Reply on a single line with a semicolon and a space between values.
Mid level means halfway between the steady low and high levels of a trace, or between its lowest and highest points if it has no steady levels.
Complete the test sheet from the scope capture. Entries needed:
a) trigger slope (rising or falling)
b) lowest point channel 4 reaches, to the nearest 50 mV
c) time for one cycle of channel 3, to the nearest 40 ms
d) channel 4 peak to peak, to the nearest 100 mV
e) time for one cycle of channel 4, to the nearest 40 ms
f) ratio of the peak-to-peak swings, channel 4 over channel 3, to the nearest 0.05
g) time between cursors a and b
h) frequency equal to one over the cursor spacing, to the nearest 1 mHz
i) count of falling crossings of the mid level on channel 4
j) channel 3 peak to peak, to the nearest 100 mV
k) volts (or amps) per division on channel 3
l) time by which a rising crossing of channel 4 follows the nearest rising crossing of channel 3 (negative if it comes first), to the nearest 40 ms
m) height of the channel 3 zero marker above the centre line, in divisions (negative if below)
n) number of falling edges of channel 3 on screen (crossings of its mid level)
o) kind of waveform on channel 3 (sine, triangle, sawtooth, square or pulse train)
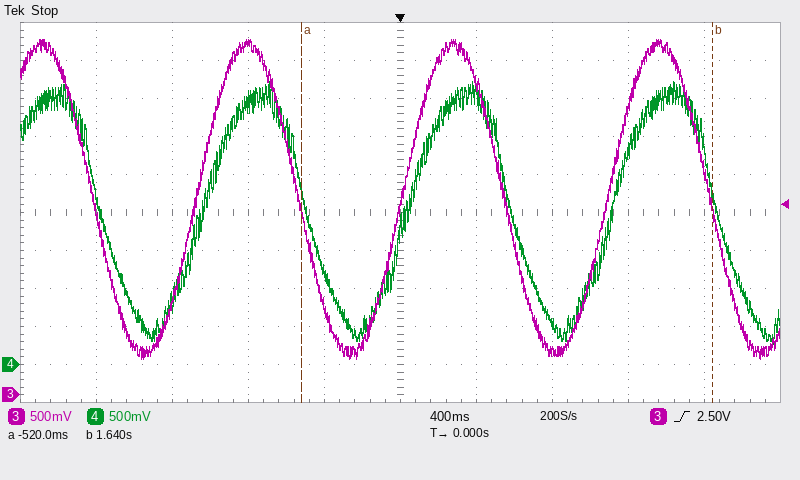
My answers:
rising; 300 mV; 1.08 s; 3.40 V; 1.08 s; 0.80; 2.16 s; 463 mHz; 4; 4.20 V; 500 mV; +40 ms; -4.8 div; 4; sine
